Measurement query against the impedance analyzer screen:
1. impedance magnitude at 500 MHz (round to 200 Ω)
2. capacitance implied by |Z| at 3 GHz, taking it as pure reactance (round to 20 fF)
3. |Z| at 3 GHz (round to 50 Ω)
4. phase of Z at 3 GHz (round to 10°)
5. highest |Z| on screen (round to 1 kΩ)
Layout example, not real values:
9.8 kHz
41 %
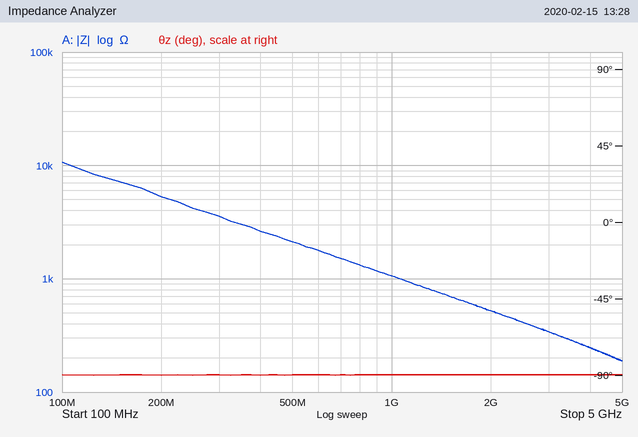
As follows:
2.2 kΩ
160 fF
350 Ω
-90°
11 kΩ
